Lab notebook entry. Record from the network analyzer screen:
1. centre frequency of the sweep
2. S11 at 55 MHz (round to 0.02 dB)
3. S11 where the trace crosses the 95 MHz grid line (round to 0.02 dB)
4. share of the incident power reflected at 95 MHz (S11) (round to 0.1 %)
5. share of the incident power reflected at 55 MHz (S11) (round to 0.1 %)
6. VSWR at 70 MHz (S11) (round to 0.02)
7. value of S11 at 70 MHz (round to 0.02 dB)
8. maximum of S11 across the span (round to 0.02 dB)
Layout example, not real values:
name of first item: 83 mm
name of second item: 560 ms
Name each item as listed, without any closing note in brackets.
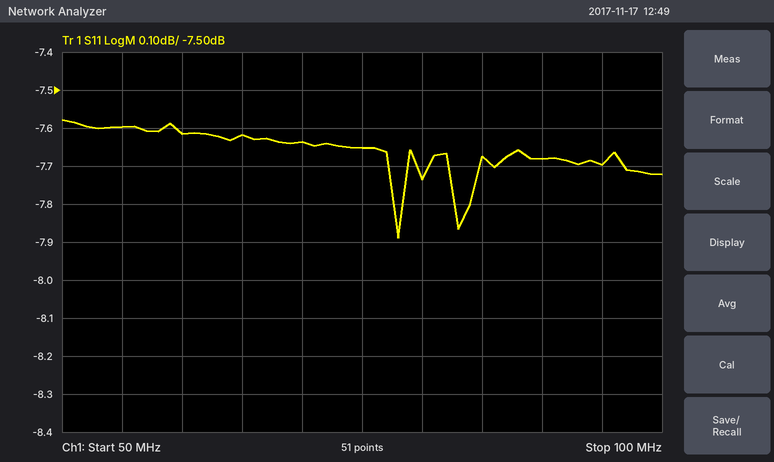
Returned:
centre frequency of the sweep: 75 MHz
S11 at 55 MHz: -7.60 dB
S11 where the trace crosses the 95 MHz grid line: -7.70 dB
share of the incident power reflected at 95 MHz (S11): 17.0 %
share of the incident power reflected at 55 MHz (S11): 17.4 %
VSWR at 70 MHz (S11): 2.42
value of S11 at 70 MHz: -7.64 dB
maximum of S11 across the span: -7.58 dB
